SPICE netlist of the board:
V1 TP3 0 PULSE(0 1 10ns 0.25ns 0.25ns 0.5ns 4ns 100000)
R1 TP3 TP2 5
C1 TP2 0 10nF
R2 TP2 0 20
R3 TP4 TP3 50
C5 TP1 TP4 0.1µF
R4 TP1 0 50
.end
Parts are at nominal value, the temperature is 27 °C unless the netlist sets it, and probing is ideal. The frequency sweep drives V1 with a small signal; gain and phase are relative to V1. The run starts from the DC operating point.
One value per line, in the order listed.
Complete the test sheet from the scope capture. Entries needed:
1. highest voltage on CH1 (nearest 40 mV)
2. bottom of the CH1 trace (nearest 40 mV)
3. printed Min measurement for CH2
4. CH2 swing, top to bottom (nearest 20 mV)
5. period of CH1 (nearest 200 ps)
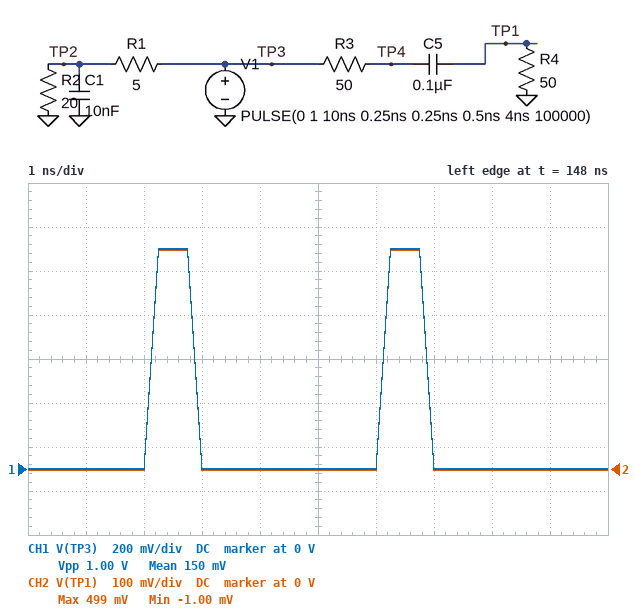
1.00 V
0 V
-1.00 mV
500 mV
4.0 ns
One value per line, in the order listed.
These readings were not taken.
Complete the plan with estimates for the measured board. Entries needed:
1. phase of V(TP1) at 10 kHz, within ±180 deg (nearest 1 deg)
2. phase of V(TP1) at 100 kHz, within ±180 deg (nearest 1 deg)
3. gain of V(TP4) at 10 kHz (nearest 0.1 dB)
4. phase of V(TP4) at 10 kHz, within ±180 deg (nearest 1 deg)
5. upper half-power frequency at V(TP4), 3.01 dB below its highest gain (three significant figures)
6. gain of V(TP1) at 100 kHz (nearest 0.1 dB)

58 deg
9 deg
-1.0 dB
-15 deg
22.5 kHz
-6.1 dB
